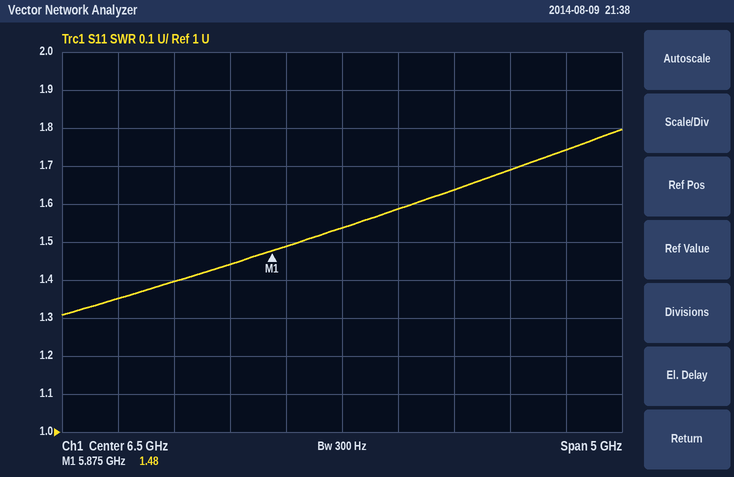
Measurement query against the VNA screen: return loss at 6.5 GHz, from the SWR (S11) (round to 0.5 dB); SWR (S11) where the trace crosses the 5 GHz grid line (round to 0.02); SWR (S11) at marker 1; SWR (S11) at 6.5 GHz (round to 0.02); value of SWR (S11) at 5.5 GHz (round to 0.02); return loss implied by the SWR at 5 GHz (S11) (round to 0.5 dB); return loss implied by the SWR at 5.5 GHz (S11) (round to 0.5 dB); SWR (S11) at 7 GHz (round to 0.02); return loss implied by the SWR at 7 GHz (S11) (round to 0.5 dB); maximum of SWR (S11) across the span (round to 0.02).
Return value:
13.5 dB
1.40
1.48
1.54
1.44
15.5 dB
15.0 dB
1.58
13.0 dB
1.80
